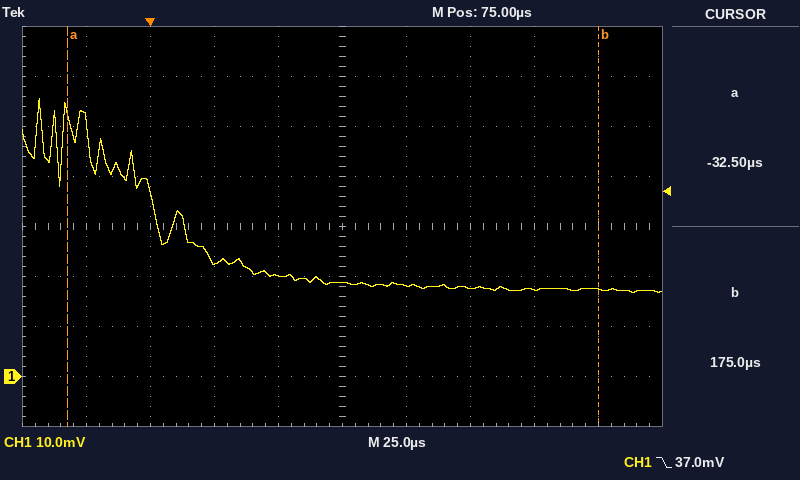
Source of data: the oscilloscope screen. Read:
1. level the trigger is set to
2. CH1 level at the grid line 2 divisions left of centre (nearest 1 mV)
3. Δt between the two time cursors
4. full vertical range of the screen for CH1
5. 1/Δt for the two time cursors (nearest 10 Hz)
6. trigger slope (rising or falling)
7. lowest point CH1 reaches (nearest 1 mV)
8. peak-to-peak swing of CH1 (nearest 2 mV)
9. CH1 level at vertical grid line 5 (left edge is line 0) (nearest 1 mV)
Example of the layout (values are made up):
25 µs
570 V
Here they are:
37.0 mV
23 mV
207.5 µs
80 mV
4.82 kHz
falling
17 mV
38 mV
19 mV
